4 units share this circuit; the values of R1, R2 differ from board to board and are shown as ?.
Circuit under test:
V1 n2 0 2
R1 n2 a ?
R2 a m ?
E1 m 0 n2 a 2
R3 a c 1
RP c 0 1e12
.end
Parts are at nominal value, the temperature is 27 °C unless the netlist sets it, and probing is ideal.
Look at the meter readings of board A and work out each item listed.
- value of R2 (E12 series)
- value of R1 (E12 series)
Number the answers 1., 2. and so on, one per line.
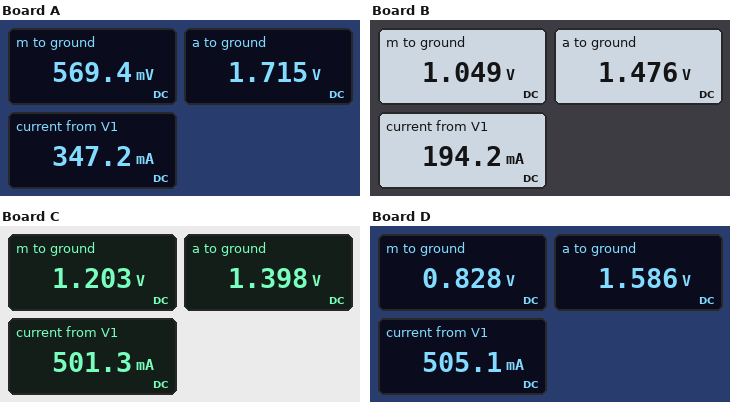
1. 3.3 Ω
2. 0.82 Ω
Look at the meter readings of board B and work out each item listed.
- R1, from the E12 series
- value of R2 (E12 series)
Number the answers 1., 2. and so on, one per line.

1. 2.7 Ω
2. 2.2 Ω
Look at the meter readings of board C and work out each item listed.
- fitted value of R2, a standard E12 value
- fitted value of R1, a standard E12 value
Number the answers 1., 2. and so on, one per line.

1. 0.39 Ω
2. 1.2 Ω
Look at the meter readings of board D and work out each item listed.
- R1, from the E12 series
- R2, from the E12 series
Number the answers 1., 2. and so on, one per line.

1. 0.82 Ω
2. 1.5 Ω
